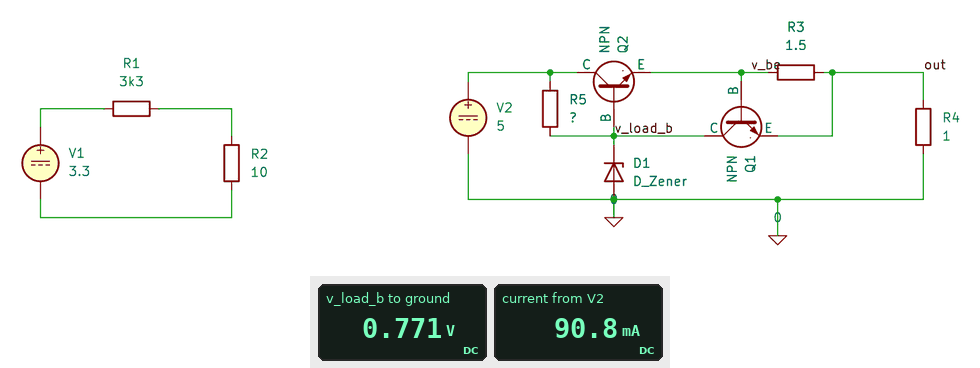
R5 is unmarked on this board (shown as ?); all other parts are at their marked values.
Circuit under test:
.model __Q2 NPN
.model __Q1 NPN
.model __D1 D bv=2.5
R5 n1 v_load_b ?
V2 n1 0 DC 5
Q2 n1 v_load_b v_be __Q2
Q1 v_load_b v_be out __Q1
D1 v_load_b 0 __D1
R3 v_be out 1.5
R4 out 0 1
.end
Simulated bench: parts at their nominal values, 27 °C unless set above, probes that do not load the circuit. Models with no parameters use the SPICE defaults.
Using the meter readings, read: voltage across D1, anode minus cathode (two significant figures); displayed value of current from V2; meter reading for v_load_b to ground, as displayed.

770 mV
90.8 mA
0.771 V
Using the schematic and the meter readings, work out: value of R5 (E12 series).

47 Ω
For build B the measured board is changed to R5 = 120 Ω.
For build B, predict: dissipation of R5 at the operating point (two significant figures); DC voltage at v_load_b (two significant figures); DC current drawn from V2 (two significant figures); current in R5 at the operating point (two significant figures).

150 mW
750 mV
36 mA
35 mA
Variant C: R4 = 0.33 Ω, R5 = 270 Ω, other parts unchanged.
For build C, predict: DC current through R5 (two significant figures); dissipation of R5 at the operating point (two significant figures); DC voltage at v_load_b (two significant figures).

16 mA
68 mW
730 mV
